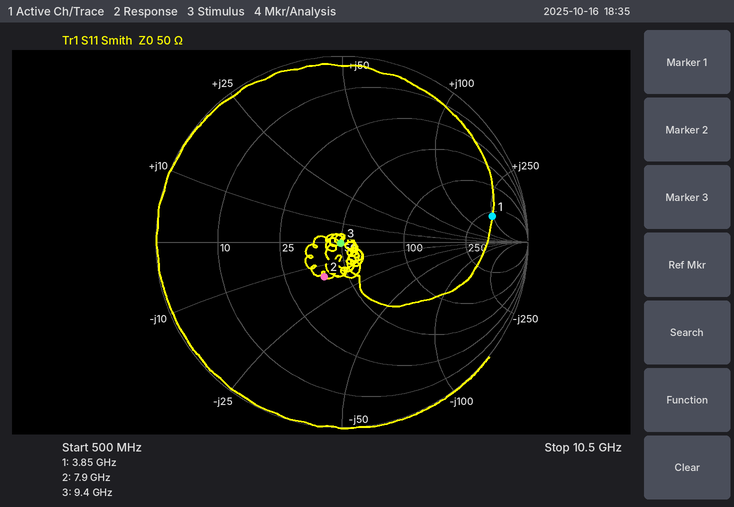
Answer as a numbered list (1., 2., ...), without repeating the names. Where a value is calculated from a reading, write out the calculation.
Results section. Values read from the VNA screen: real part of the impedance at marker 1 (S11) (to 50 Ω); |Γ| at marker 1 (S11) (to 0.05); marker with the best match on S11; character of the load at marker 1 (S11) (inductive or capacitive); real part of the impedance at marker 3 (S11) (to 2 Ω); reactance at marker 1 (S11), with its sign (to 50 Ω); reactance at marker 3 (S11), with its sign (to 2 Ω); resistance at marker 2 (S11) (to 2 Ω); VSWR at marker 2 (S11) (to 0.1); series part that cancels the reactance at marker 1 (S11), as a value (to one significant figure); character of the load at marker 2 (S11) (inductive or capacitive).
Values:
1. 300 Ω
2. 0.80
3. marker 3
4. inductive
5. 50 Ω
6. +250 Ω
7. 0 Ω
8. 38 Ω
9. 1.5
10. C = 1/(2π × 3.85 GHz × 250 Ω) ≈ 165 fF, so 200 fF to one significant figure
11. capacitive
